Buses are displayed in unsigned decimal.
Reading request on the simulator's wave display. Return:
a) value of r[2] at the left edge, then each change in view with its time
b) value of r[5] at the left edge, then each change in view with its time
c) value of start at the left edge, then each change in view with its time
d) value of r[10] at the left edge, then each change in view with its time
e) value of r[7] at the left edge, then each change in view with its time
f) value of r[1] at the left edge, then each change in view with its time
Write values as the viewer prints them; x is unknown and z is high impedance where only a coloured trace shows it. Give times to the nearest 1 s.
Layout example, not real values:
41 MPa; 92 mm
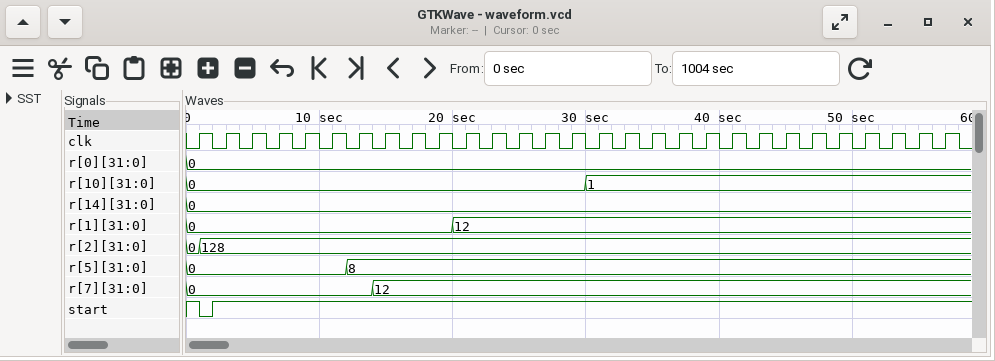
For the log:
0, 128 at 1 s; 0, 8 at 12 s; 1, 0 at 1 s, 1 at 2 s; 0, 1 at 30 s; 0, 12 at 14 s; 0, 12 at 20 s
